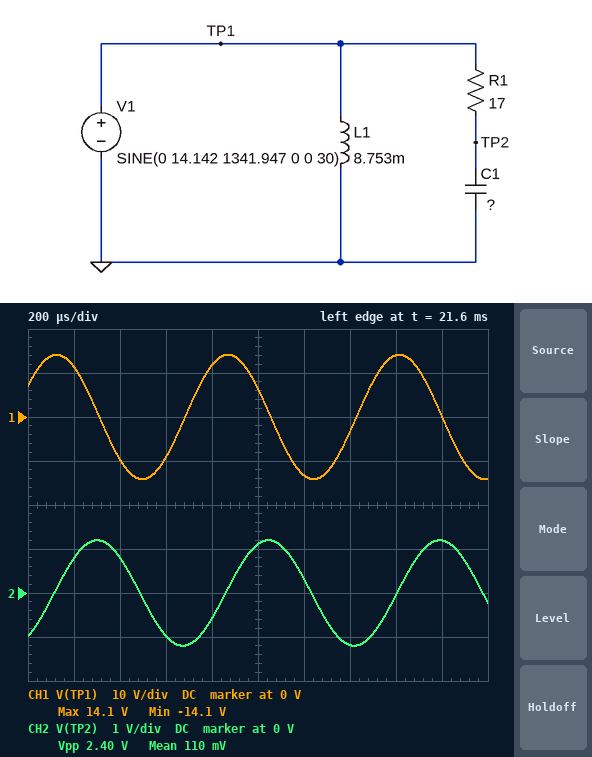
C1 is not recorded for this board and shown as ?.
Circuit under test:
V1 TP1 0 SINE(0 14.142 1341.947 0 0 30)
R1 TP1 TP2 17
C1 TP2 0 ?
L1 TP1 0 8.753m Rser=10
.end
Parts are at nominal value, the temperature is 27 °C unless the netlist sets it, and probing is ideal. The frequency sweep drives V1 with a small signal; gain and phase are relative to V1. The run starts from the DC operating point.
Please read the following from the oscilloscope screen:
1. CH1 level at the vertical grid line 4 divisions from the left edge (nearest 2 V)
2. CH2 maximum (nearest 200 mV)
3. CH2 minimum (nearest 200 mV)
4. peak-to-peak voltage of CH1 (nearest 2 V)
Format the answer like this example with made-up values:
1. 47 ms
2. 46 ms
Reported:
1. 12 V
2. 1.2 V
3. -1.2 V
4. 28 V
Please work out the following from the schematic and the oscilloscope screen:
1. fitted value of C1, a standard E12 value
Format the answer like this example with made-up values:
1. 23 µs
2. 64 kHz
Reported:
1. 82 µF
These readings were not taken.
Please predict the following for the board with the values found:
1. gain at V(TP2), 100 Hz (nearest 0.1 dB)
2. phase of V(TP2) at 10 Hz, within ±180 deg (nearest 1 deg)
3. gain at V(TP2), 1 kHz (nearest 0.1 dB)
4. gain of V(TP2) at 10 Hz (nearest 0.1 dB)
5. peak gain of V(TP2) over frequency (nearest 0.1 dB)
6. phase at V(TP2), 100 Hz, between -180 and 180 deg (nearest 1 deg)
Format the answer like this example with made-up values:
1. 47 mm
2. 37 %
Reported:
1. -2.5 dB
2. -5 deg
3. -18.9 dB
4. 0 dB
5. 0 dB
6. -41 deg
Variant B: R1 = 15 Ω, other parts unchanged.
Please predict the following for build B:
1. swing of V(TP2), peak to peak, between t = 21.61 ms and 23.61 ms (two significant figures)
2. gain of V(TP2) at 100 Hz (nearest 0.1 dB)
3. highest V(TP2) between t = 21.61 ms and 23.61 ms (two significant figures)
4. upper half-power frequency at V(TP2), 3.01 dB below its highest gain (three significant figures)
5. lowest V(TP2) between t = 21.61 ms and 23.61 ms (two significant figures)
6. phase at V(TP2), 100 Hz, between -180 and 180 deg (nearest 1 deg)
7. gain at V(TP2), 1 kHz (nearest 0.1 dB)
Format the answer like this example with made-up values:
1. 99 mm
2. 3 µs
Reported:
1. 2.7 V
2. -2.0 dB
3. 1.4 V
4. 129 Hz
5. -1.4 V
6. -38 deg
7. -17.8 dB
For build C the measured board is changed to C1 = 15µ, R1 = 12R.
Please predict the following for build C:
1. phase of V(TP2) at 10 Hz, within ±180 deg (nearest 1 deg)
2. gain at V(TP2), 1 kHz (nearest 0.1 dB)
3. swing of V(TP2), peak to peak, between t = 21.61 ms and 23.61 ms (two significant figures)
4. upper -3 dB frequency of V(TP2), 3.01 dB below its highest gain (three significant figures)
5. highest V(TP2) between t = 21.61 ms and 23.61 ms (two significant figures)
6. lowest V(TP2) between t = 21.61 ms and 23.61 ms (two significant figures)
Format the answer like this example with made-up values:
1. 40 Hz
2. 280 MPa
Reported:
1. -1 deg
2. -3.6 dB
3. 16 V
4. 884 Hz
5. 7.8 V
6. -7.8 V
